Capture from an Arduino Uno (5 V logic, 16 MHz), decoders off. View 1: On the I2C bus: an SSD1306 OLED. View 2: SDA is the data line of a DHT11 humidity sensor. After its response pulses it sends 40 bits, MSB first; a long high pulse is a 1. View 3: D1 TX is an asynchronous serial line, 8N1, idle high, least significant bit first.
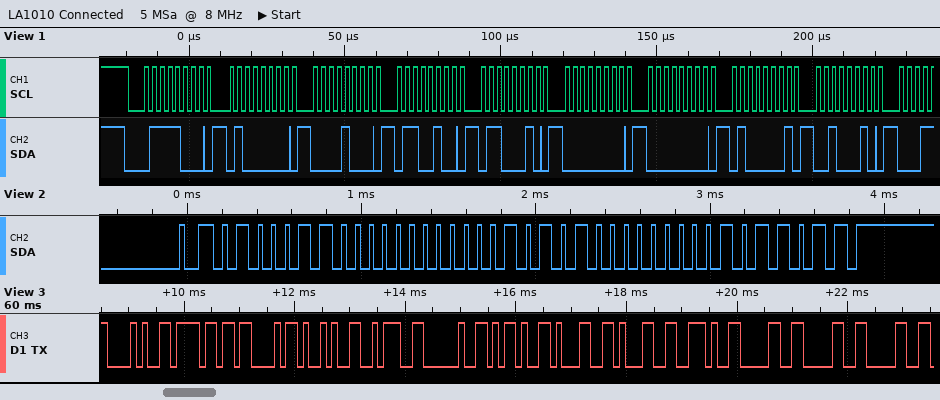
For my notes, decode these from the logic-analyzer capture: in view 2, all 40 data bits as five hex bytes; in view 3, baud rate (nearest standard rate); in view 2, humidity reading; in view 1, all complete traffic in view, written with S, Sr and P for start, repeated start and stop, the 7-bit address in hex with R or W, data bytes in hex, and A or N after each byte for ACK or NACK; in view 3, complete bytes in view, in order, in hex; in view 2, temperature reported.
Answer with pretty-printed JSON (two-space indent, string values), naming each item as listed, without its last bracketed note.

{
  "in view 2, all 40 data bits as five hex bytes": "46 00 15 00 5B",
  "in view 3, baud rate": "9600 baud",
  "in view 2, humidity reading": "70 %",
  "in view 1, all complete traffic in view, written with S, Sr and P for start, repeated start and stop, the 7-bit address in hex with R or W, data bytes in hex, and A or N after each byte for ACK or NACK": "S 3CW A 40 A 08 A 64 A 62 A 00 A 00 A 41 A 22 A",
  "in view 3, complete bytes in view, in order, in hex": "0x28 0x6F 0x43 0x29 0x3A 0x20 0x2D 0x31 0x31 0x2E 0x30 0x30 0x30",
  "in view 2, temperature reported": "21.0 °C"
}
